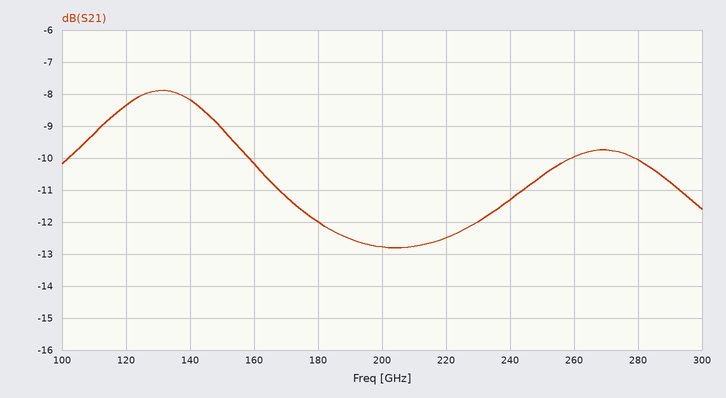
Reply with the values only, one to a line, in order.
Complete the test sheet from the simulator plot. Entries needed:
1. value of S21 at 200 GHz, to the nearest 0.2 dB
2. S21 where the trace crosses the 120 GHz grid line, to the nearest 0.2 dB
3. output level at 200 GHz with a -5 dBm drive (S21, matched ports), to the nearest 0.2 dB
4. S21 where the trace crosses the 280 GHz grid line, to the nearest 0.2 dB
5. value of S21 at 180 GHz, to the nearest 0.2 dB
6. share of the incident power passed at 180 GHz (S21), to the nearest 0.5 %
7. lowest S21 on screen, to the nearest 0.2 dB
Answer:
-12.8 dB
-8.4 dB
-17.8 dBm
-10.0 dB
-12.0 dB
6.5 %
-12.8 dB
